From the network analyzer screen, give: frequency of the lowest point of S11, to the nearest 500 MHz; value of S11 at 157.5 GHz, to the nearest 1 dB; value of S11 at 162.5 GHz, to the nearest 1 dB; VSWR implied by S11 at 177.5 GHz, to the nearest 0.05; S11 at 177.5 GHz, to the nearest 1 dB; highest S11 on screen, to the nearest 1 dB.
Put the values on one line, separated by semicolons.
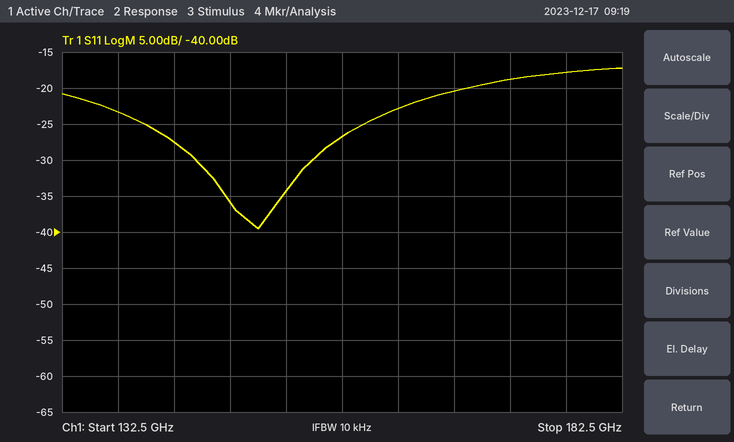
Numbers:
150.0 GHz; -27 dB; -23 dB; 1.30; -18 dB; -17 dB
